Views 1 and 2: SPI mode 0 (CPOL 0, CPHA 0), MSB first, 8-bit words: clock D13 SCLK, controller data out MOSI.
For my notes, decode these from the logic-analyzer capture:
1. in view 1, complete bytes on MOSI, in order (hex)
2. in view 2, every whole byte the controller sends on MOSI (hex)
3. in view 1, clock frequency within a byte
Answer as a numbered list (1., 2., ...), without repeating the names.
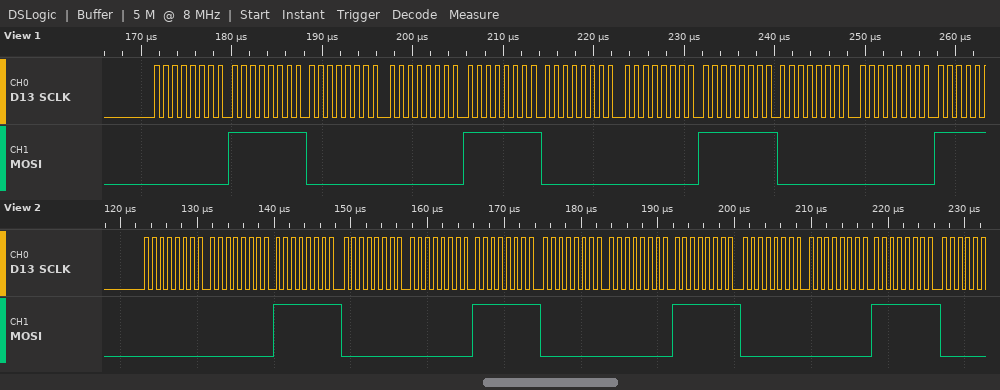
1. 00 FF 00 00 FF 00 00 FF 00 00
2. 00 00 FF 00 00 FF 00 00 FF 00 00 FF
3. 1 MHz
